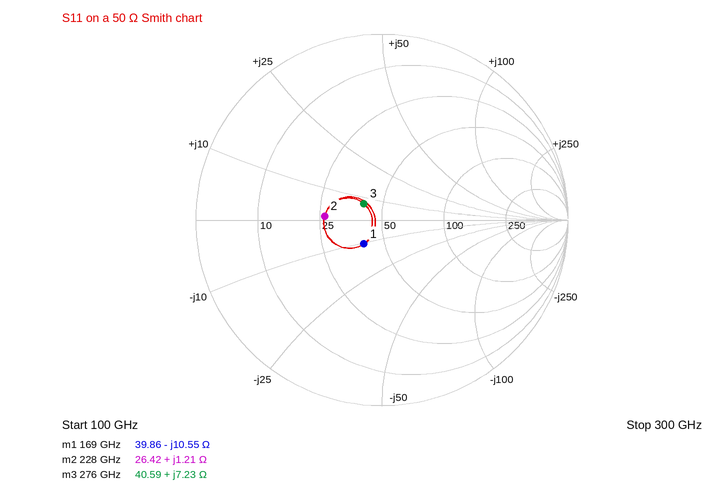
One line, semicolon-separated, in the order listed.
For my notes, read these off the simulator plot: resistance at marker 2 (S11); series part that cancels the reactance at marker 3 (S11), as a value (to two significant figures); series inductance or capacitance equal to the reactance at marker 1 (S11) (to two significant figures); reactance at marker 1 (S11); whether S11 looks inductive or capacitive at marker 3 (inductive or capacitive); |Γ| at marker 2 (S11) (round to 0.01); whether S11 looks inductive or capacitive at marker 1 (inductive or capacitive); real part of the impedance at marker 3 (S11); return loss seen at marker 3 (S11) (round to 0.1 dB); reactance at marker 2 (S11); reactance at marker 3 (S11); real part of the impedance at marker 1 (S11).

26.42 Ω; 80 fF; 89 fF; -10.55 Ω; inductive; 0.31; capacitive; 40.59 Ω; 17.7 dB; +1.21 Ω; +7.23 Ω; 39.86 Ω
